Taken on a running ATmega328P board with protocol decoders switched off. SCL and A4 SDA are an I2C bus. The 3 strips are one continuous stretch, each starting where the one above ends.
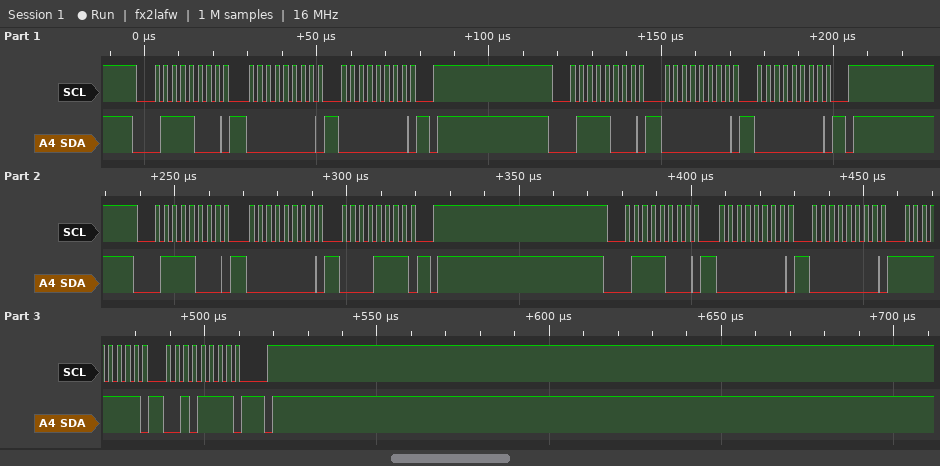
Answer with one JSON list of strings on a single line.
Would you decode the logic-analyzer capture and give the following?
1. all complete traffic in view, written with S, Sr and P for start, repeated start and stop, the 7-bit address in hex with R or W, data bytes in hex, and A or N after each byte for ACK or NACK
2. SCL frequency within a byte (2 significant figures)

["S 3CW A 00 A 00 A P S 3CW A 00 A 00 A P S 3CW A 00 A 0F A P S 3CW A 00 A 00 A FF A 2F A P", "400 kHz"]
